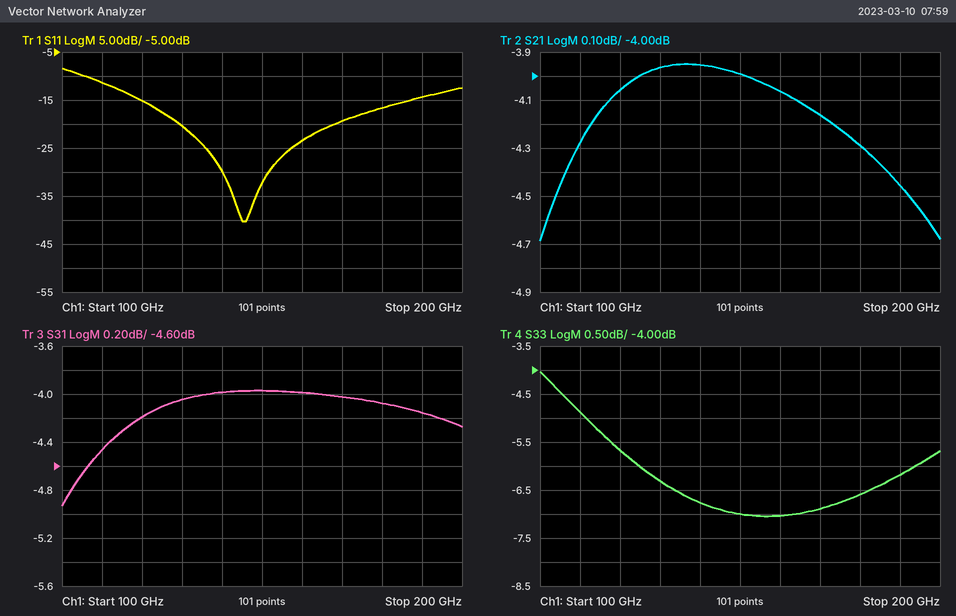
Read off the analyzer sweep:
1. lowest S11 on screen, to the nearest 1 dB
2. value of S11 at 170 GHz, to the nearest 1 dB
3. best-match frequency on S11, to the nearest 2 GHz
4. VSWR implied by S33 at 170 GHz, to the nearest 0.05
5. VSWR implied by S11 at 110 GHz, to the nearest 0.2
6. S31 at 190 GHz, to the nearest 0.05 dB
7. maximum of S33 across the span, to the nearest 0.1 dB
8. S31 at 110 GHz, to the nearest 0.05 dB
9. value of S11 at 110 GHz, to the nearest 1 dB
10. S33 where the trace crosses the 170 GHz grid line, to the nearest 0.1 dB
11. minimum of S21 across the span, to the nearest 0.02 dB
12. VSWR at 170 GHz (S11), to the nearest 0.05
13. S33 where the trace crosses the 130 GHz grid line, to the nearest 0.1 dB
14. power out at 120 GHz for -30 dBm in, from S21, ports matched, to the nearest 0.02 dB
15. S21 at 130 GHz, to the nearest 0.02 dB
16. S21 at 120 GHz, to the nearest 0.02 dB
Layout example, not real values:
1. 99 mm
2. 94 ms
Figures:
1. -40 dB
2. -19 dB
3. 146 GHz
4. 2.65
5. 1.8
6. -4.15 dB
7. -4.0 dB
8. -4.45 dB
9. -11 dB
10. -6.9 dB
11. -4.68 dB
12. 1.25
13. -6.3 dB
14. -34.06 dBm
15. -3.96 dB
16. -4.06 dB
